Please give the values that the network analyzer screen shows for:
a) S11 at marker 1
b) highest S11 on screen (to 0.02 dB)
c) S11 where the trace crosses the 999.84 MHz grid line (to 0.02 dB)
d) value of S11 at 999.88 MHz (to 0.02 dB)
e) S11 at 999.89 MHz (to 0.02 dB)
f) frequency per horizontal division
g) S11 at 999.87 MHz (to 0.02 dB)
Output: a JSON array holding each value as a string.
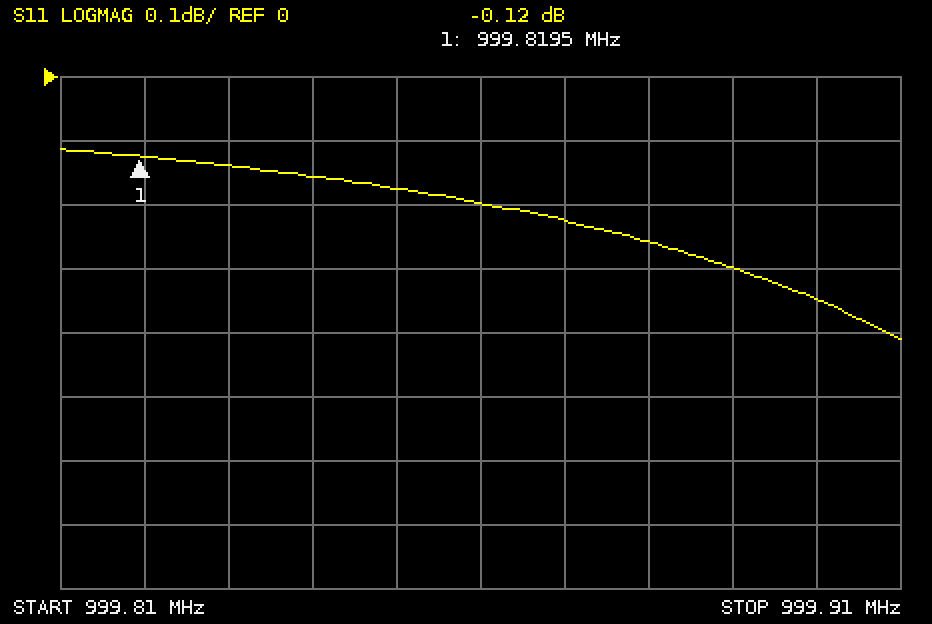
["-0.12 dB", "-0.12 dB", "-0.16 dB", "-0.26 dB", "-0.30 dB", "10 kHz", "-0.22 dB"]
